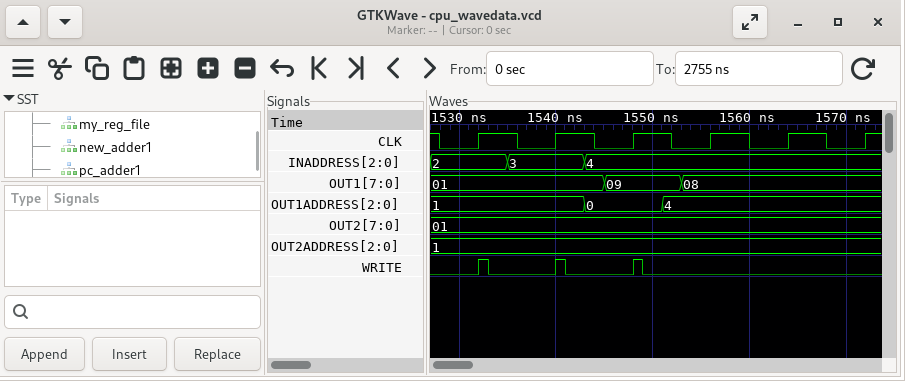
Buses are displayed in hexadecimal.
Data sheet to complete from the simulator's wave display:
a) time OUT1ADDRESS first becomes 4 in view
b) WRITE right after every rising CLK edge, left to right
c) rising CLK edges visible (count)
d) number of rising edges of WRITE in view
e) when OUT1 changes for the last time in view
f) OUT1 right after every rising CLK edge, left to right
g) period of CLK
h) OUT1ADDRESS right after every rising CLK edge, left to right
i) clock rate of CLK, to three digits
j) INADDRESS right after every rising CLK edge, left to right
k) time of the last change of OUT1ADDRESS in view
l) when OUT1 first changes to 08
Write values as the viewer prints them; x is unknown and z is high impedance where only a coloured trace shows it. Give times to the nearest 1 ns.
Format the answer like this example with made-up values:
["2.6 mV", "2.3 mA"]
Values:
["1551 ns", "1 1 1 0 0 0", "6", "3", "1553 ns", "01, 01, 09, 08, 08, 08", "8 ns", "1, 1, 0, 4, 4, 4", "125 MHz", "2, 3, 4, 4, 4, 4", "1551 ns", "1553 ns"]
